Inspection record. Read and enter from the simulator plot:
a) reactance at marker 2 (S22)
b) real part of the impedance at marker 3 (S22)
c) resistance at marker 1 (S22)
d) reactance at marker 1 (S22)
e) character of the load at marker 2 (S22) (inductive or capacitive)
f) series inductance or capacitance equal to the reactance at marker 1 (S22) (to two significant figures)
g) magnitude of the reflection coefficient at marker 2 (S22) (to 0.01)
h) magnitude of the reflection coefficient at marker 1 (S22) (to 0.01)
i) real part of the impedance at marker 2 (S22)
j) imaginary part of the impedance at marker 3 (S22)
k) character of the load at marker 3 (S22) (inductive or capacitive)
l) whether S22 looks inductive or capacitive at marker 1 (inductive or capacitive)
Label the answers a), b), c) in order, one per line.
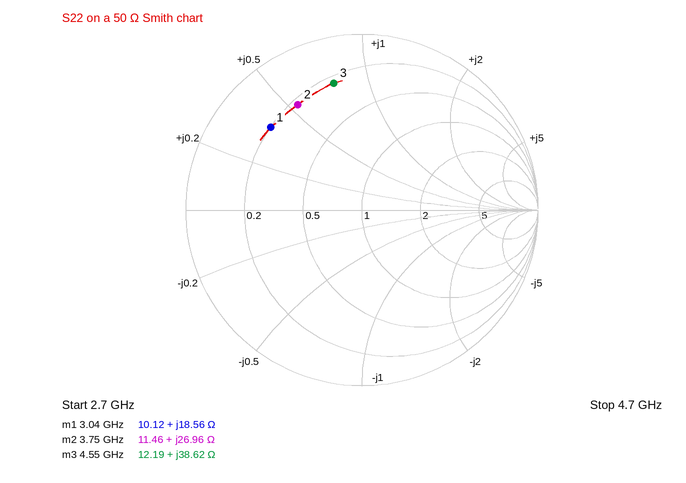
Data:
a) +26.96 Ω
b) 12.19 Ω
c) 10.12 Ω
d) +18.56 Ω
e) inductive
f) 970 pH
g) 0.70
h) 0.70
i) 11.46 Ω
j) +38.62 Ω
k) inductive
l) inductive
